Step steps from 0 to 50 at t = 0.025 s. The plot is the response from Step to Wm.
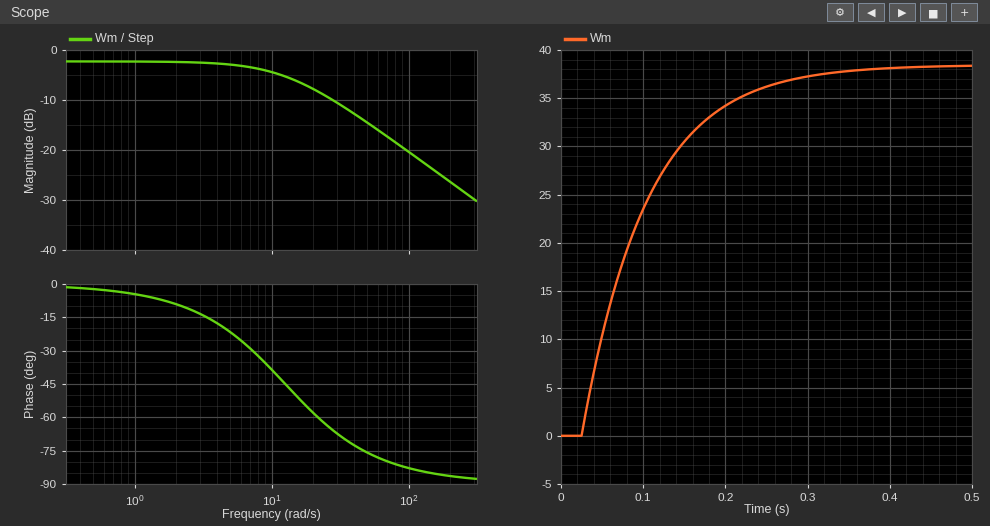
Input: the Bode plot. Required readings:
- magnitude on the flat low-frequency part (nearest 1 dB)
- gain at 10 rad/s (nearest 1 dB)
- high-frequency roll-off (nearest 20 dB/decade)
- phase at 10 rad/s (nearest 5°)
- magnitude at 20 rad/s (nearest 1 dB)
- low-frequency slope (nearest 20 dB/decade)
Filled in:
-2 dB
-4 dB
-20 dB/decade
-40°
-8 dB
0 dB/decade
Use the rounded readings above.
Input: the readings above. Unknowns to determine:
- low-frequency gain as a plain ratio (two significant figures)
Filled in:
0.79
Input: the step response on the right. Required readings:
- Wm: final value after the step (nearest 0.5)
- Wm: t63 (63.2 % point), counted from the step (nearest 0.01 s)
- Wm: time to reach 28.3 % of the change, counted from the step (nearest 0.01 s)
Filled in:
38.5
0.08 s
0.03 s
